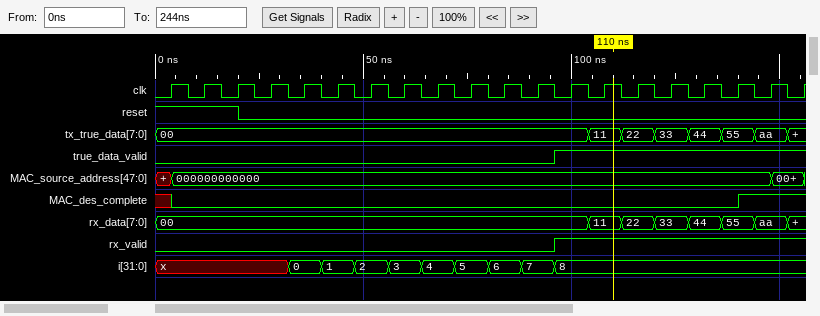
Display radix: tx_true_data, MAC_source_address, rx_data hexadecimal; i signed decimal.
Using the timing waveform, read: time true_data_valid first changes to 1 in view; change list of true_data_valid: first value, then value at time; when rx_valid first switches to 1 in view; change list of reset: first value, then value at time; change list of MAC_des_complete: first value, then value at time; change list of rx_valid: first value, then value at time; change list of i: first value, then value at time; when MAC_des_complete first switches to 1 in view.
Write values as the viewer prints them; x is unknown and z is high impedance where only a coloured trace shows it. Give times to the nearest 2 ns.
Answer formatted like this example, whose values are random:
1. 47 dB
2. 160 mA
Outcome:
1. 96 ns
2. 0, 1 at 96 ns
3. 96 ns
4. 1, 0 at 20 ns
5. x, 0 at 4 ns, 1 at 140 ns
6. 0, 1 at 96 ns
7. x, 0 at 32 ns, 1 at 40 ns, 2 at 48 ns, 3 at 56 ns, 4 at 64 ns, 5 at 72 ns, 6 at 80 ns, 7 at 88 ns, 8 at 96 ns
8. 140 ns
